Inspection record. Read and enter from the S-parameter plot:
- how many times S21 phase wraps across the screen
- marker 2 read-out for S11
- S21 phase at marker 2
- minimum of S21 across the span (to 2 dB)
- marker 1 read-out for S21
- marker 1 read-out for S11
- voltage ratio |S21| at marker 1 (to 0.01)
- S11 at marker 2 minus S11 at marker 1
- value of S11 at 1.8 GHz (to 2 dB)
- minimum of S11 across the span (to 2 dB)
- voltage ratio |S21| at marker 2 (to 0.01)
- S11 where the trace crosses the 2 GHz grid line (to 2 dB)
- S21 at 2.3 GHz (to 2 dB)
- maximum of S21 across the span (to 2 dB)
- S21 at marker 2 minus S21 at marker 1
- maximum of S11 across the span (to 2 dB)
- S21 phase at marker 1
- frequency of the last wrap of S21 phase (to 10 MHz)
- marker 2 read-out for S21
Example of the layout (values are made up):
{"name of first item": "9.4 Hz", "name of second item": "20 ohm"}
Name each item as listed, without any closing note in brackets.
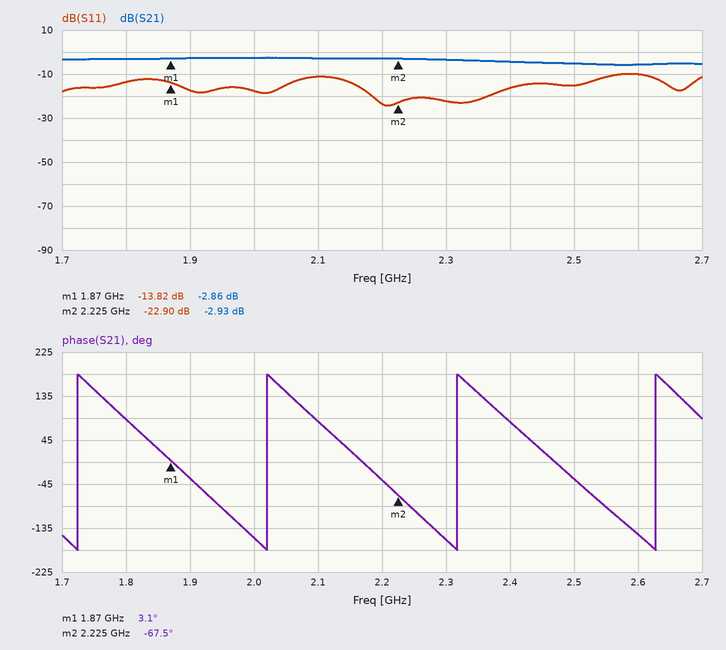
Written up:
{"how many times S21 phase wraps across the screen": "4", "marker 2 read-out for S11": "-22.90 dB", "S21 phase at marker 2": "-67.5°", "minimum of S21 across the span": "-6 dB", "marker 1 read-out for S21": "-2.86 dB", "marker 1 read-out for S11": "-13.82 dB", "voltage ratio |S21| at marker 1": "0.72", "S11 at marker 2 minus S11 at marker 1": "-9.08 dB", "value of S11 at 1.8 GHz": "-14 dB", "minimum of S11 across the span": "-24 dB", "voltage ratio |S21| at marker 2": "0.71", "S11 where the trace crosses the 2 GHz grid line": "-18 dB", "S21 at 2.3 GHz": "-4 dB", "maximum of S21 across the span": "-2 dB", "S21 at marker 2 minus S21 at marker 1": "-0.07 dB", "maximum of S11 across the span": "-10 dB", "S21 phase at marker 1": "3.1°", "frequency of the last wrap of S21 phase": "2.63 GHz", "marker 2 read-out for S21": "-2.93 dB"}
